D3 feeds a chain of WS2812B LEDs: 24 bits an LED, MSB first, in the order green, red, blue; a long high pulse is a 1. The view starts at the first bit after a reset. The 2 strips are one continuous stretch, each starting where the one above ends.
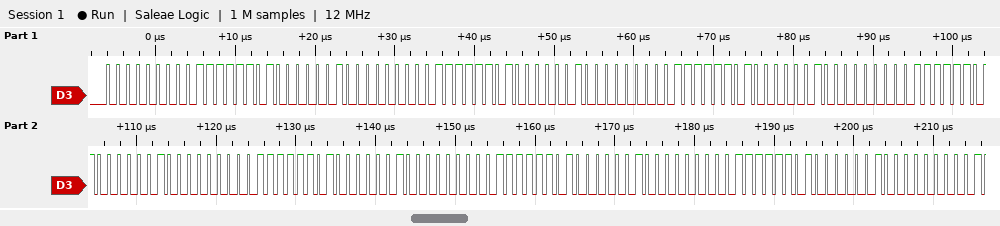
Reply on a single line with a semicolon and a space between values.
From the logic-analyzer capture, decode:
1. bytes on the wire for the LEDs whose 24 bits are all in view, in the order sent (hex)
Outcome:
00 7E 81 00 7E 81 00 7E 81 00 7E 81 00 7E 81 00 7E 81 00 7E 81
